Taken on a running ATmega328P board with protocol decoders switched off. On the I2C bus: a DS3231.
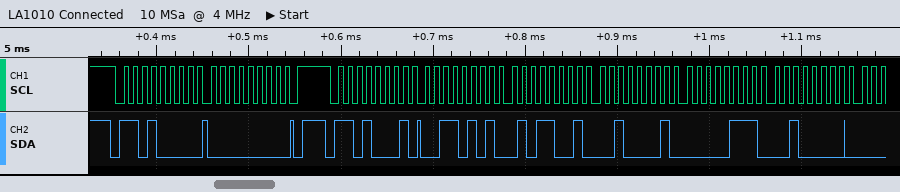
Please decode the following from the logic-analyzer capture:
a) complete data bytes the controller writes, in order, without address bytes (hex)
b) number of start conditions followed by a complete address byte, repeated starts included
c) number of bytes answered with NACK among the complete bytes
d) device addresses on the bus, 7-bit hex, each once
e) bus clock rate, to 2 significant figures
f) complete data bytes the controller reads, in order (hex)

00
2
0
0x68
100 kHz
35 59 21 07 20
